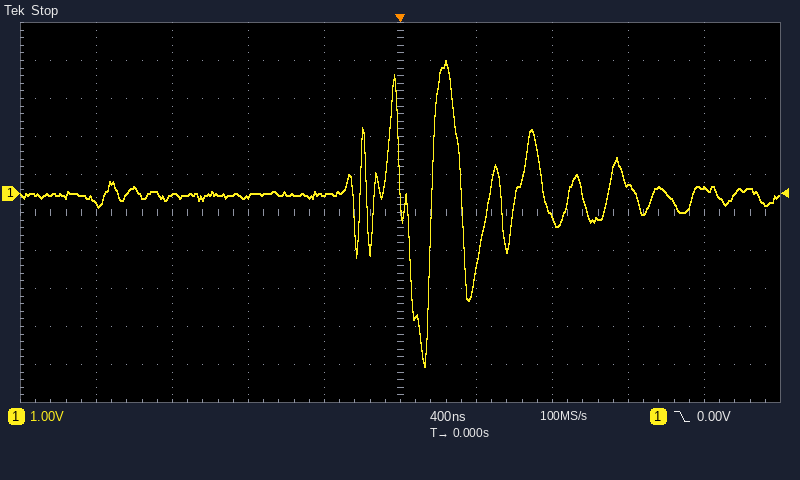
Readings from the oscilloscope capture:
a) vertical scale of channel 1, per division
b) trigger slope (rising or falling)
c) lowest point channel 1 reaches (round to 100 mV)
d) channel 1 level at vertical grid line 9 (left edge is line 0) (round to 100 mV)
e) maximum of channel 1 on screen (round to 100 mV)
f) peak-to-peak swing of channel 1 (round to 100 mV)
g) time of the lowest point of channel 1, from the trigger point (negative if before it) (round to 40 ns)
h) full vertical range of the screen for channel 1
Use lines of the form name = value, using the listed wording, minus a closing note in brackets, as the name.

vertical scale of channel 1, per division = 1 V
trigger slope = falling
lowest point channel 1 reaches = -4.6 V
channel 1 level at vertical grid line 9 (left edge is line 0) = 100 mV
maximum of channel 1 on screen = 3.5 V
peak-to-peak swing of channel 1 = 8.1 V
time of the lowest point of channel 1, from the trigger point (negative if before it) = +120 ns
full vertical range of the screen for channel 1 = 10 V
